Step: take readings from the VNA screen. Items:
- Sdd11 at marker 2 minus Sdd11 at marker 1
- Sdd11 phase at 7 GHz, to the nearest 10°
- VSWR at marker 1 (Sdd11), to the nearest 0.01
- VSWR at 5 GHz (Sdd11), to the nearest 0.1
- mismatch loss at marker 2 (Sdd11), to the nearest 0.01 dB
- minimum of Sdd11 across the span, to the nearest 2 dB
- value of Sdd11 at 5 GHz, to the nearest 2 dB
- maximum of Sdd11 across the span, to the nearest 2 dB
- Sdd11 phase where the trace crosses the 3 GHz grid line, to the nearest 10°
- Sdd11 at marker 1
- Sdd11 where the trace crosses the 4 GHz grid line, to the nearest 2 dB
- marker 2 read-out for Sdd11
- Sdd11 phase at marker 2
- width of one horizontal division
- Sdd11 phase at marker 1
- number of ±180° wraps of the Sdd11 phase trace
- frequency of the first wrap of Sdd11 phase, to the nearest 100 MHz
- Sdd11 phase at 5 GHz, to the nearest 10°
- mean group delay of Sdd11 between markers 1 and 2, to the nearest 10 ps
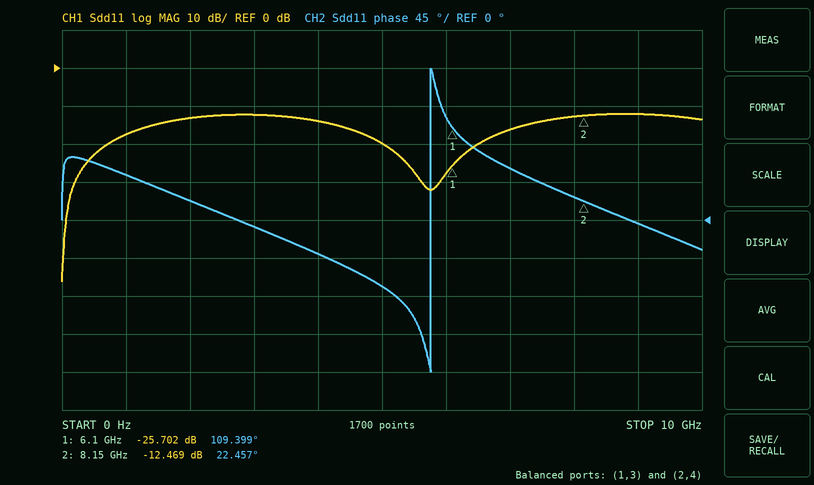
13.233 dB
60°
1.11
1.2
0.25 dB
-56 dB
-20 dB
-12 dB
-10°
-25.702 dB
-14 dB
-12.469 dB
22.457°
1 GHz
109.399°
1
5.8 GHz
-80°
120 ps
